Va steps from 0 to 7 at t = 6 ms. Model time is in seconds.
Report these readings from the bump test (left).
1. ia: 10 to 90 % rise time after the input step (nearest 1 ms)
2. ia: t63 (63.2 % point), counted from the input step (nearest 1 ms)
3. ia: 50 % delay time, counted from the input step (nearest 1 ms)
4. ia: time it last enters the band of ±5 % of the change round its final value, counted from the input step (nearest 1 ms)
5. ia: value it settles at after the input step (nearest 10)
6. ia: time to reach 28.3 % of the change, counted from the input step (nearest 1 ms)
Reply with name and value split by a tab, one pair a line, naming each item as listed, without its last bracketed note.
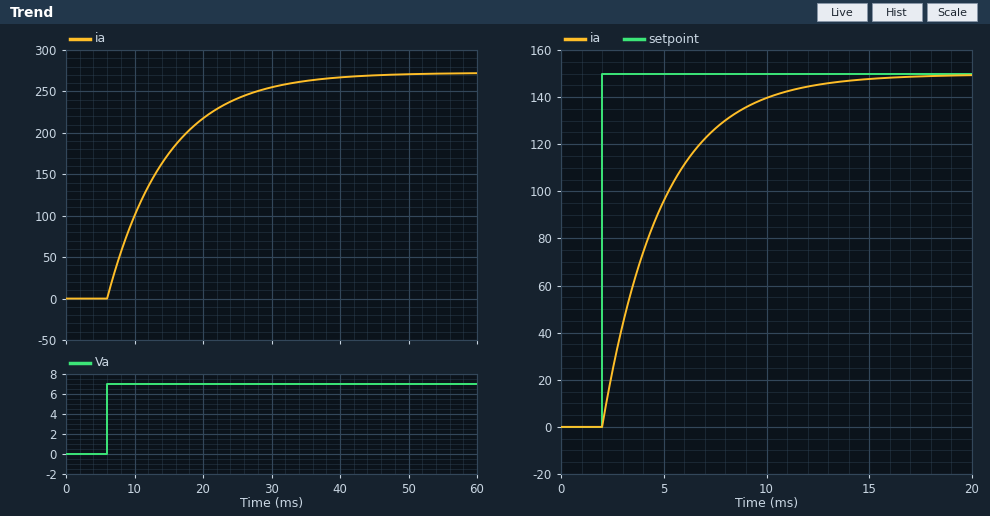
ia: 10 to 90 % rise time after the input step	19 ms
ia: t63 (63.2 % point), counted from the input step	9 ms
ia: 50 % delay time, counted from the input step	6 ms
ia: time it last enters the band of ±5 % of the change round its final value, counted from the input step	26 ms
ia: value it settles at after the input step	270
ia: time to reach 28.3 % of the change, counted from the input step	3 ms
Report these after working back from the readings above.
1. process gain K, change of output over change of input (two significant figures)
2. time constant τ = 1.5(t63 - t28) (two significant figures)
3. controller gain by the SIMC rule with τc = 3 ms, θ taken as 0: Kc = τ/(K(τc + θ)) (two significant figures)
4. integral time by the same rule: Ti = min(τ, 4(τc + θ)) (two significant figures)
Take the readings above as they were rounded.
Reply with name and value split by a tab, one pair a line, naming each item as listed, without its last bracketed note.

process gain K, change of output over change of input	39
time constant τ = 1.5(t63 - t28)	9.0 ms
controller gain by the SIMC rule with τc = 3 ms, θ taken as 0: Kc = τ/(K(τc + θ))	0.077
integral time by the same rule: Ti = min(τ, 4(τc + θ))	9.0 ms
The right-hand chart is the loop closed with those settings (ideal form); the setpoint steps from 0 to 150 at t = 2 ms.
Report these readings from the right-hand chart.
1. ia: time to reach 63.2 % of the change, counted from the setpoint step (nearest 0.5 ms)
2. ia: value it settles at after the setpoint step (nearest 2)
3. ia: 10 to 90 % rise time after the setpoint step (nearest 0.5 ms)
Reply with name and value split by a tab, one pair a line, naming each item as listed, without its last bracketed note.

ia: time to reach 63.2 % of the change, counted from the setpoint step	3.0 ms
ia: value it settles at after the setpoint step	150
ia: 10 to 90 % rise time after the setpoint step	6.5 ms
